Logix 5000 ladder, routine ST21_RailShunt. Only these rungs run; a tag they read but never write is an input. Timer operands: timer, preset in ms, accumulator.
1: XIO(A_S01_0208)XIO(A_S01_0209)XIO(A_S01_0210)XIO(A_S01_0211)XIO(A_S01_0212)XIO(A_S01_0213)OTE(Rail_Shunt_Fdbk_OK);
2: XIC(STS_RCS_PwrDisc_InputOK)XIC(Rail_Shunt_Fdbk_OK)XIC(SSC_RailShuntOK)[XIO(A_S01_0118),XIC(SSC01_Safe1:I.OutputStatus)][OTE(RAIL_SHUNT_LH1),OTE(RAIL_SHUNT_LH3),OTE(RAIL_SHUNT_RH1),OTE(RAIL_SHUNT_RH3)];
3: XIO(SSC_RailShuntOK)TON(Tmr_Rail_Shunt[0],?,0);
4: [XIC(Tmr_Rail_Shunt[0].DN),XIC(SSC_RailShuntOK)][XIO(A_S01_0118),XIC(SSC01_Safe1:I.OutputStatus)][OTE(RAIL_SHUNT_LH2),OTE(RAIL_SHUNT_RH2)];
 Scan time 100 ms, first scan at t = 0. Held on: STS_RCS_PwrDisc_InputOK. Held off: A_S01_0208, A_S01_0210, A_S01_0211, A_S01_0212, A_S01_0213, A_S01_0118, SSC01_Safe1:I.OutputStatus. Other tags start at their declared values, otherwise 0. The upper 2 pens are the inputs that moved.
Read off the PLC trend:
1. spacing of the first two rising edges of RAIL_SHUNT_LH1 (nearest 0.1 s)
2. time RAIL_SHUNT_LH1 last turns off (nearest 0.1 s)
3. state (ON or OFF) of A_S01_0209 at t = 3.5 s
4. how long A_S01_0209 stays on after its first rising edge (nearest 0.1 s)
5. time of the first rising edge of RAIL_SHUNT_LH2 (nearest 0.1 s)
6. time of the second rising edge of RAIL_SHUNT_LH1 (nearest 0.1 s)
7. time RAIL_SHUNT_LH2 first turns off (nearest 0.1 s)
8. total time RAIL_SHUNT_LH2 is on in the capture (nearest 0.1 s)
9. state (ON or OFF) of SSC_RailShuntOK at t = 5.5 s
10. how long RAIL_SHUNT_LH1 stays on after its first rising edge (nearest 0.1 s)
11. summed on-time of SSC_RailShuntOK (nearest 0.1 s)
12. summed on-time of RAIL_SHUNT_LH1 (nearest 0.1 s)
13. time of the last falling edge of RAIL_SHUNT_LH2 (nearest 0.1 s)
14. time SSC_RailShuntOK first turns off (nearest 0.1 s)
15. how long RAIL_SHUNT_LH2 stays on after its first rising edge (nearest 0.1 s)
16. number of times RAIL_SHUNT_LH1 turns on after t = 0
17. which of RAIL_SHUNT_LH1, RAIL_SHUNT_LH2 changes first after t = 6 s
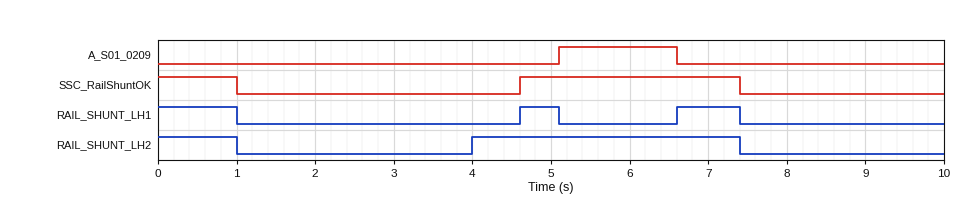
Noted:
2.0 s
7.4 s
OFF
1.5 s
4.0 s
6.6 s
1.0 s
4.4 s
ON
0.5 s
3.8 s
2.3 s
7.4 s
1.0 s
3.4 s
2
RAIL_SHUNT_LH1
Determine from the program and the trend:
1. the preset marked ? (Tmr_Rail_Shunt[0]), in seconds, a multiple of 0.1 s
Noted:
3.0 s
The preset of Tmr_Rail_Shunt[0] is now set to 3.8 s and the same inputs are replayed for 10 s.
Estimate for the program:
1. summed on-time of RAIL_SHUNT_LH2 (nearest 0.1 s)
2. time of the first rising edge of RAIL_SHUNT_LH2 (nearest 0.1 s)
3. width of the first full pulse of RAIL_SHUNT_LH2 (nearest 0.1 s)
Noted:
3.8 s
4.6 s
2.8 s
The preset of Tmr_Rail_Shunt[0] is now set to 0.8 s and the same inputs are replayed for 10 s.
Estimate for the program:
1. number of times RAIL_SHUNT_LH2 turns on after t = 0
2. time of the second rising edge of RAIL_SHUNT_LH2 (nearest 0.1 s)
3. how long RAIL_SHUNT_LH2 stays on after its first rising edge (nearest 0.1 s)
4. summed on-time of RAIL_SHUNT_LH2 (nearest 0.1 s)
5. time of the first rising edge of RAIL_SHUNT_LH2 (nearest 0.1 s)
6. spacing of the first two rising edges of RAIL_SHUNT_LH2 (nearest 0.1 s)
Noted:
2
8.2 s
5.6 s
8.4 s
1.8 s
6.4 s
